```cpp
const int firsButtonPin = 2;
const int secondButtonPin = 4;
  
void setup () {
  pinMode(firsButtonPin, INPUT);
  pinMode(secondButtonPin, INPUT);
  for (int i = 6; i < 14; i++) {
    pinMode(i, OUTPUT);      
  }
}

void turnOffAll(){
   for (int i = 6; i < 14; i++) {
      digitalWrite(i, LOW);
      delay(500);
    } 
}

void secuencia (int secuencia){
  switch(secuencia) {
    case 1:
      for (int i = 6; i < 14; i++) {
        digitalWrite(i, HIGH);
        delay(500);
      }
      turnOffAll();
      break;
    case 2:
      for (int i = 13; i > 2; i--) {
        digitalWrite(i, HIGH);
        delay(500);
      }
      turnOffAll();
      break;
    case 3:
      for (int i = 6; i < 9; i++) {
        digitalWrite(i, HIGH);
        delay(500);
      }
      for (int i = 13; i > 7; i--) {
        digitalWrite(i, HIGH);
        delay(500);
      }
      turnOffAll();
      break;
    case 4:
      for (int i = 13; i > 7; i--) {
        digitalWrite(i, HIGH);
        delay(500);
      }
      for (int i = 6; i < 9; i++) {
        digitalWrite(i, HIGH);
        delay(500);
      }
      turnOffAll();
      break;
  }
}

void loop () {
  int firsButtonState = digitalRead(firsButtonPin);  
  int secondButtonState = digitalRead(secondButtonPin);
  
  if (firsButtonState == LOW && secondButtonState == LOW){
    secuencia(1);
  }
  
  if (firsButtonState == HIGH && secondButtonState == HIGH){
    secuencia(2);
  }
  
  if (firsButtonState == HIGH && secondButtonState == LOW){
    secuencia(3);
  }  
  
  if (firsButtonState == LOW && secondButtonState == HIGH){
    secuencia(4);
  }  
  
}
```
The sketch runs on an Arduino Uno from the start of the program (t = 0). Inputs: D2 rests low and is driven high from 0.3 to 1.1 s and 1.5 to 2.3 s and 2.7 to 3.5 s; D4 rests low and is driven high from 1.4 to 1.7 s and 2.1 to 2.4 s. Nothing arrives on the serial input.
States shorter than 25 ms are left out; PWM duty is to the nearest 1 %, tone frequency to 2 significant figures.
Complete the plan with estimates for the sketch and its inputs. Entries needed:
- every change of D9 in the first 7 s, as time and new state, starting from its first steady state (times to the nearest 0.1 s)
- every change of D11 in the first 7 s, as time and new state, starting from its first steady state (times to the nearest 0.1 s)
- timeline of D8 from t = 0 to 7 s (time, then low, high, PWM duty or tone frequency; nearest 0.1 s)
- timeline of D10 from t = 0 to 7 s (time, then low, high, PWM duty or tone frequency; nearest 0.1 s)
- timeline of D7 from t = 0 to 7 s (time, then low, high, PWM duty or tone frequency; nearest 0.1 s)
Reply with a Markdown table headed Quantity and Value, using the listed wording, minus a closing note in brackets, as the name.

| Quantity | Value |
|---|---|
| every change of D9 in the first 7 s, as time and new state, starting from its first steady state | 0 s low; 1.5 s high; 5.5 s low |
| every change of D11 in the first 7 s, as time and new state, starting from its first steady state | 0 s low; 2.5 s high; 6.5 s low |
| timeline of D8 from t = 0 to 7 s | 0 s low; 1 s high; 5 s low |
| timeline of D10 from t = 0 to 7 s | 0 s low; 2 s high; 6 s low |
| timeline of D7 from t = 0 to 7 s | 0 s low; 0.5 s high; 4.5 s low |
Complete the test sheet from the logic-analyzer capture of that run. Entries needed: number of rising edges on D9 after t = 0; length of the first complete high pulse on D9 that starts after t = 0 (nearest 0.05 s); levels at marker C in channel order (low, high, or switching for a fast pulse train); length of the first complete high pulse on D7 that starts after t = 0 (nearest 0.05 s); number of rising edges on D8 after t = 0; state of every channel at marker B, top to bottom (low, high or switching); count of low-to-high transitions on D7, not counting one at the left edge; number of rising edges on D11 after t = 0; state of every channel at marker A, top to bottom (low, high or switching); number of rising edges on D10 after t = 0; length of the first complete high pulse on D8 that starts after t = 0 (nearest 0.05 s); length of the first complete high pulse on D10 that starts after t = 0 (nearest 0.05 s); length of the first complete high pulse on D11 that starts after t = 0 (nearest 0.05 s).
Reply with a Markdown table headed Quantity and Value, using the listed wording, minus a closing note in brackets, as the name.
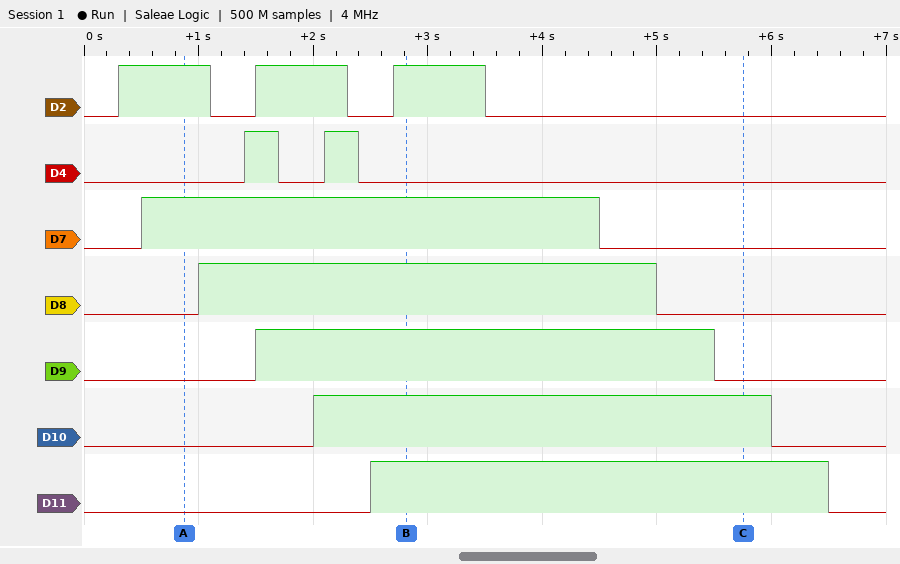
| Quantity | Value |
|---|---|
| number of rising edges on D9 after t = 0 | 1 |
| length of the first complete high pulse on D9 that starts after t = 0 | 4.00 s |
| levels at marker C in channel order | D2 low, D4 low, D7 low, D8 low, D9 low, D10 high, D11 high |
| length of the first complete high pulse on D7 that starts after t = 0 | 4.00 s |
| number of rising edges on D8 after t = 0 | 1 |
| state of every channel at marker B, top to bottom | D2 high, D4 low, D7 high, D8 high, D9 high, D10 high, D11 high |
| count of low-to-high transitions on D7, not counting one at the left edge | 1 |
| number of rising edges on D11 after t = 0 | 1 |
| state of every channel at marker A, top to bottom | D2 high, D4 low, D7 high, D8 low, D9 low, D10 low, D11 low |
| number of rising edges on D10 after t = 0 | 1 |
| length of the first complete high pulse on D8 that starts after t = 0 | 4.00 s |
| length of the first complete high pulse on D10 that starts after t = 0 | 4.00 s |
| length of the first complete high pulse on D11 that starts after t = 0 | 4.00 s |
